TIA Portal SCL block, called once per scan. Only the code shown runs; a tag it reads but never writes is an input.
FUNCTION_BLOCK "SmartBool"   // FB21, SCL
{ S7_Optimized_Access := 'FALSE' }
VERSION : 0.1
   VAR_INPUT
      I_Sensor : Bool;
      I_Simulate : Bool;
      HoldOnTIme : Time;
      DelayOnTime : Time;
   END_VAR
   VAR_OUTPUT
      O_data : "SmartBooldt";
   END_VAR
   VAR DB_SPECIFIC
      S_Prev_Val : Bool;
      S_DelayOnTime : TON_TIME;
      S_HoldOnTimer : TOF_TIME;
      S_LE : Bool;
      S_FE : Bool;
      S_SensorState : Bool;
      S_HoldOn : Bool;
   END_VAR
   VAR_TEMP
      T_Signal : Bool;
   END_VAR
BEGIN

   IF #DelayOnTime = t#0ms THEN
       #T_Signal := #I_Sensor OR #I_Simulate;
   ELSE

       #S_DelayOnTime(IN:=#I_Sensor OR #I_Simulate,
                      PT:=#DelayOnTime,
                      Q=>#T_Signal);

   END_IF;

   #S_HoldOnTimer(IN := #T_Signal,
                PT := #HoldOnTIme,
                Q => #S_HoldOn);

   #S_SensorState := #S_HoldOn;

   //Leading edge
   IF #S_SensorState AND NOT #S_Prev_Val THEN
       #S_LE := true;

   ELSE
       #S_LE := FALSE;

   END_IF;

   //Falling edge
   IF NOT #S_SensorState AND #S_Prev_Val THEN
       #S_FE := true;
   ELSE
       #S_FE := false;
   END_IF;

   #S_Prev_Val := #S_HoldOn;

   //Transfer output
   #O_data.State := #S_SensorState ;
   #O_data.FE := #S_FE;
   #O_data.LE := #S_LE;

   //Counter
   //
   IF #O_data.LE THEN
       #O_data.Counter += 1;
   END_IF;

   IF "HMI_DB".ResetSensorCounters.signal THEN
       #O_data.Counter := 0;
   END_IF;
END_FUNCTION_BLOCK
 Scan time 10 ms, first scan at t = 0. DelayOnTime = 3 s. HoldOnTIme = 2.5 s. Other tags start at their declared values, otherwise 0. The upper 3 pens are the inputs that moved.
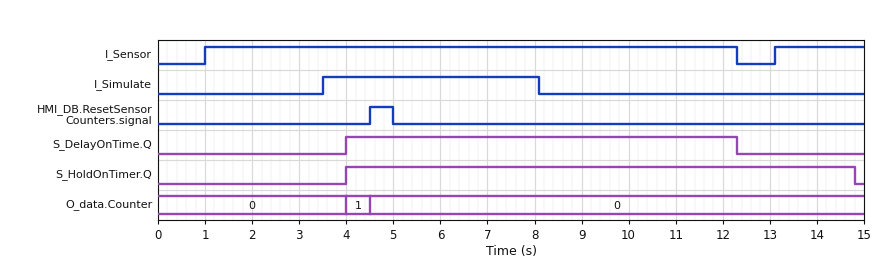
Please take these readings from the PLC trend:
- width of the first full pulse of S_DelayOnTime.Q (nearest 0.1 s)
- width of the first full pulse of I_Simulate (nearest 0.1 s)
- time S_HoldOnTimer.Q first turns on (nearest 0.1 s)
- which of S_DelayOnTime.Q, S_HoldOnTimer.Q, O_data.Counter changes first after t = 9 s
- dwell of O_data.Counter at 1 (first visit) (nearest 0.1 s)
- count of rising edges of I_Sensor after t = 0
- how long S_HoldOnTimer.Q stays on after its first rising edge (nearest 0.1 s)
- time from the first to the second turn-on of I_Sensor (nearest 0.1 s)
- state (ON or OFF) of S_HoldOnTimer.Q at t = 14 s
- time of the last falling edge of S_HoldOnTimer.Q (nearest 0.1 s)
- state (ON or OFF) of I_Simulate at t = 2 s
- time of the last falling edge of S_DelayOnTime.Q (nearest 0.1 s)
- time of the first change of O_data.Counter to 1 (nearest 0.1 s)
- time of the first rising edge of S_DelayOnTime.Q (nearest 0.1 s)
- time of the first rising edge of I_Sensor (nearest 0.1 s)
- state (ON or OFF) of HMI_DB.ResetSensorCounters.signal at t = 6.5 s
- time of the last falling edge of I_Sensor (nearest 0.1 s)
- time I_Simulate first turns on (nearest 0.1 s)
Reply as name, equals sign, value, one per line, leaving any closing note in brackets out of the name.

width of the first full pulse of S_DelayOnTime.Q = 8.3 s
width of the first full pulse of I_Simulate = 4.6 s
time S_HoldOnTimer.Q first turns on = 4.0 s
which of S_DelayOnTime.Q, S_HoldOnTimer.Q, O_data.Counter changes first after t = 9 s = S_DelayOnTime.Q
dwell of O_data.Counter at 1 (first visit) = 0.5 s
count of rising edges of I_Sensor after t = 0 = 2
how long S_HoldOnTimer.Q stays on after its first rising edge = 10.8 s
time from the first to the second turn-on of I_Sensor = 12.1 s
state (ON or OFF) of S_HoldOnTimer.Q at t = 14 s = ON
time of the last falling edge of S_HoldOnTimer.Q = 14.8 s
state (ON or OFF) of I_Simulate at t = 2 s = OFF
time of the last falling edge of S_DelayOnTime.Q = 12.3 s
time of the first change of O_data.Counter to 1 = 4.0 s
time of the first rising edge of S_DelayOnTime.Q = 4.0 s
time of the first rising edge of I_Sensor = 1.0 s
state (ON or OFF) of HMI_DB.ResetSensorCounters.signal at t = 6.5 s = OFF
time of the last falling edge of I_Sensor = 12.3 s
time I_Simulate first turns on = 3.5 s
